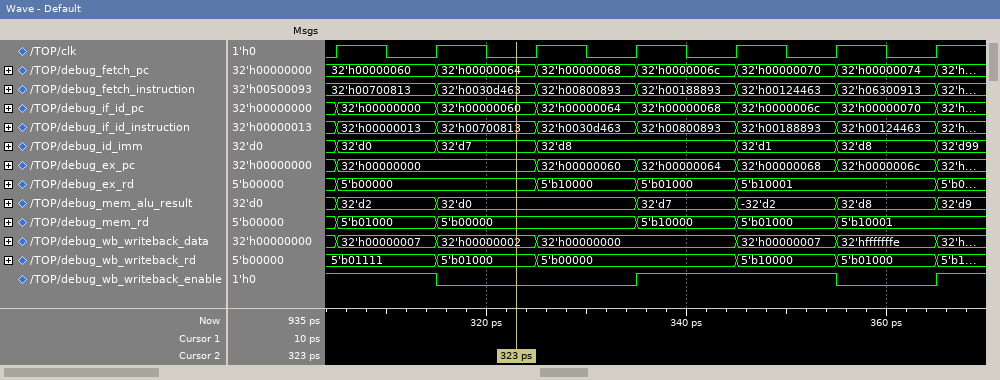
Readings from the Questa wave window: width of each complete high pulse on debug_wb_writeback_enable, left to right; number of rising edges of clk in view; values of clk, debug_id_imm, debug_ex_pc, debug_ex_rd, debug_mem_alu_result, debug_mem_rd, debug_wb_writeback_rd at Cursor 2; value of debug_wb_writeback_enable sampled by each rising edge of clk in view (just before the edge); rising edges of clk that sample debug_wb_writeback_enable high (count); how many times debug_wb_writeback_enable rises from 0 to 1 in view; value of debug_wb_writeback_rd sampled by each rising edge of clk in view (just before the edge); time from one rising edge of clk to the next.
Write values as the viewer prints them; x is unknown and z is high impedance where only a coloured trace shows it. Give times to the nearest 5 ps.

20 ps
7
clk=0, debug_id_imm=32'd7, debug_ex_pc=32'h00000000, debug_ex_rd=5'b00000, debug_mem_alu_result=32'd0, debug_mem_rd=5'b00000, debug_wb_writeback_rd=5'b01000
1 1 0 0 1 1 0
4
2
5'b01111, 5'b01111, 5'b01000, 5'b00000, 5'b00000, 5'b10000, 5'b01000
10 ps
